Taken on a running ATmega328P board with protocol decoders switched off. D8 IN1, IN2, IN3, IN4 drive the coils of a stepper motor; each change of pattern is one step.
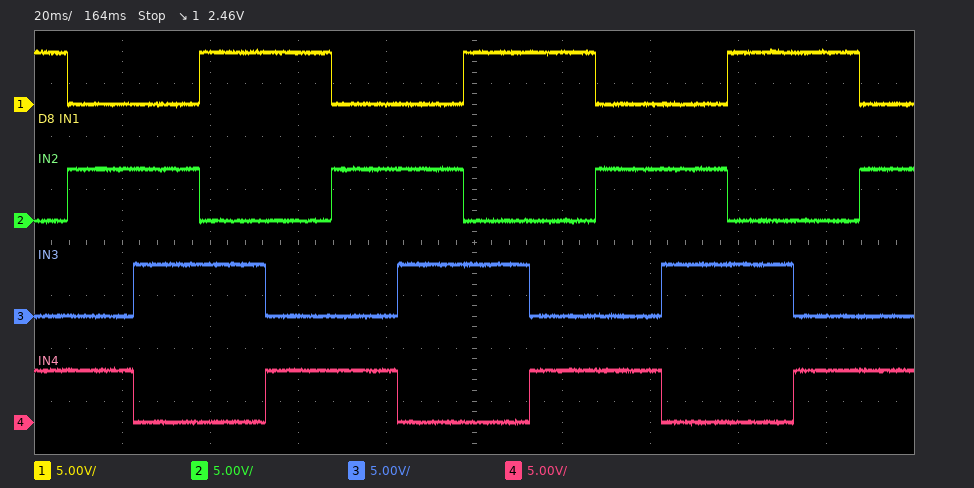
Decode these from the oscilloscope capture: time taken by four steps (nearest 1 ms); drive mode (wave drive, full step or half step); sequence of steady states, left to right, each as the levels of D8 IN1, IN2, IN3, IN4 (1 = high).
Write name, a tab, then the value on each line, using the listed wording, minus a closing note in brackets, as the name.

time taken by four steps	60 ms
drive mode	full step
sequence of steady states, left to right, each as the levels of D8 IN1, IN2, IN3, IN4	1001 0101 0110 1010 1001 0101 0110 1010 1001 0101 0110 1010 1001 0101
